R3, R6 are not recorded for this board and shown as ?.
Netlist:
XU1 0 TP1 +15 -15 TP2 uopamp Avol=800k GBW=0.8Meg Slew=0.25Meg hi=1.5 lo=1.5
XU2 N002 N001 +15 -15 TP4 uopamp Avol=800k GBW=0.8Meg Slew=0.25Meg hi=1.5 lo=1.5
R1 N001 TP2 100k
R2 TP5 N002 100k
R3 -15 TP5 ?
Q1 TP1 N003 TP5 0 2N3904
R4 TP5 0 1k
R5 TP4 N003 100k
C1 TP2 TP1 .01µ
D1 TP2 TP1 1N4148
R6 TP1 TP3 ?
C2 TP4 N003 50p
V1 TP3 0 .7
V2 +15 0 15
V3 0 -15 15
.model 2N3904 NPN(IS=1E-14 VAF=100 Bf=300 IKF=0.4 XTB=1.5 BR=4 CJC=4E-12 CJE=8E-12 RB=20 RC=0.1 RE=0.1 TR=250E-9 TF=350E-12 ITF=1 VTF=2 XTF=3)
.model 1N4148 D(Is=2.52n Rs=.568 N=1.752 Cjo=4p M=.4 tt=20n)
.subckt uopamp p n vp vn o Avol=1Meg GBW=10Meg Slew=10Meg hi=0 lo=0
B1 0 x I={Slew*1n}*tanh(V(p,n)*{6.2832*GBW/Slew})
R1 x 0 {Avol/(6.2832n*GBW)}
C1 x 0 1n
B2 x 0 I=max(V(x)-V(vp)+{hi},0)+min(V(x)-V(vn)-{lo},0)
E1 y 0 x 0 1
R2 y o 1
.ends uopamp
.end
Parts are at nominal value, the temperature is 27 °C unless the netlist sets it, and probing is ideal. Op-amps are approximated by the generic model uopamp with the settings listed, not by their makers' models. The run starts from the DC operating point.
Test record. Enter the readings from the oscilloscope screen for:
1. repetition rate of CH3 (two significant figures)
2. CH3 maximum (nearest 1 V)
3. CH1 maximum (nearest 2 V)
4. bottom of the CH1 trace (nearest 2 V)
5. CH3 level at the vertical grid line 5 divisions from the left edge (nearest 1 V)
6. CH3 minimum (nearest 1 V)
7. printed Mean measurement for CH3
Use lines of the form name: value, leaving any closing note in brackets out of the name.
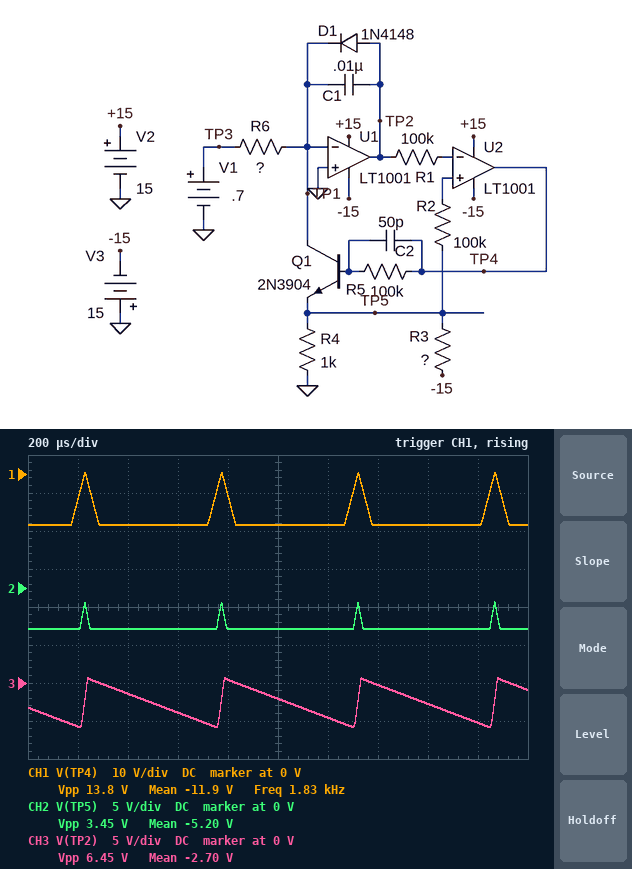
repetition rate of CH3: 1.8 kHz
CH3 maximum: 1 V
CH1 maximum: 0 V
bottom of the CH1 trace: -14 V
CH3 level at the vertical grid line 5 divisions from the left edge: -2 V
CH3 minimum: -6 V
printed Mean measurement for CH3: -2.70 V
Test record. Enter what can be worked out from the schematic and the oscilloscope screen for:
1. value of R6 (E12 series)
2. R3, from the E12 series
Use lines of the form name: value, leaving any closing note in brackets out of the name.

value of R6: 5.6 kΩ
R3, from the E12 series: 1.8 kΩ
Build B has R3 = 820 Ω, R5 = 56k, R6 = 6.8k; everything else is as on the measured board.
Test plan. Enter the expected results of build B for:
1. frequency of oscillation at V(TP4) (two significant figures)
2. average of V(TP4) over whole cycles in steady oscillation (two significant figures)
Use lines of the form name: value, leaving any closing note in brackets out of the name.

frequency of oscillation at V(TP4): 1.1 kHz
average of V(TP4) over whole cycles in steady oscillation: -13 V
